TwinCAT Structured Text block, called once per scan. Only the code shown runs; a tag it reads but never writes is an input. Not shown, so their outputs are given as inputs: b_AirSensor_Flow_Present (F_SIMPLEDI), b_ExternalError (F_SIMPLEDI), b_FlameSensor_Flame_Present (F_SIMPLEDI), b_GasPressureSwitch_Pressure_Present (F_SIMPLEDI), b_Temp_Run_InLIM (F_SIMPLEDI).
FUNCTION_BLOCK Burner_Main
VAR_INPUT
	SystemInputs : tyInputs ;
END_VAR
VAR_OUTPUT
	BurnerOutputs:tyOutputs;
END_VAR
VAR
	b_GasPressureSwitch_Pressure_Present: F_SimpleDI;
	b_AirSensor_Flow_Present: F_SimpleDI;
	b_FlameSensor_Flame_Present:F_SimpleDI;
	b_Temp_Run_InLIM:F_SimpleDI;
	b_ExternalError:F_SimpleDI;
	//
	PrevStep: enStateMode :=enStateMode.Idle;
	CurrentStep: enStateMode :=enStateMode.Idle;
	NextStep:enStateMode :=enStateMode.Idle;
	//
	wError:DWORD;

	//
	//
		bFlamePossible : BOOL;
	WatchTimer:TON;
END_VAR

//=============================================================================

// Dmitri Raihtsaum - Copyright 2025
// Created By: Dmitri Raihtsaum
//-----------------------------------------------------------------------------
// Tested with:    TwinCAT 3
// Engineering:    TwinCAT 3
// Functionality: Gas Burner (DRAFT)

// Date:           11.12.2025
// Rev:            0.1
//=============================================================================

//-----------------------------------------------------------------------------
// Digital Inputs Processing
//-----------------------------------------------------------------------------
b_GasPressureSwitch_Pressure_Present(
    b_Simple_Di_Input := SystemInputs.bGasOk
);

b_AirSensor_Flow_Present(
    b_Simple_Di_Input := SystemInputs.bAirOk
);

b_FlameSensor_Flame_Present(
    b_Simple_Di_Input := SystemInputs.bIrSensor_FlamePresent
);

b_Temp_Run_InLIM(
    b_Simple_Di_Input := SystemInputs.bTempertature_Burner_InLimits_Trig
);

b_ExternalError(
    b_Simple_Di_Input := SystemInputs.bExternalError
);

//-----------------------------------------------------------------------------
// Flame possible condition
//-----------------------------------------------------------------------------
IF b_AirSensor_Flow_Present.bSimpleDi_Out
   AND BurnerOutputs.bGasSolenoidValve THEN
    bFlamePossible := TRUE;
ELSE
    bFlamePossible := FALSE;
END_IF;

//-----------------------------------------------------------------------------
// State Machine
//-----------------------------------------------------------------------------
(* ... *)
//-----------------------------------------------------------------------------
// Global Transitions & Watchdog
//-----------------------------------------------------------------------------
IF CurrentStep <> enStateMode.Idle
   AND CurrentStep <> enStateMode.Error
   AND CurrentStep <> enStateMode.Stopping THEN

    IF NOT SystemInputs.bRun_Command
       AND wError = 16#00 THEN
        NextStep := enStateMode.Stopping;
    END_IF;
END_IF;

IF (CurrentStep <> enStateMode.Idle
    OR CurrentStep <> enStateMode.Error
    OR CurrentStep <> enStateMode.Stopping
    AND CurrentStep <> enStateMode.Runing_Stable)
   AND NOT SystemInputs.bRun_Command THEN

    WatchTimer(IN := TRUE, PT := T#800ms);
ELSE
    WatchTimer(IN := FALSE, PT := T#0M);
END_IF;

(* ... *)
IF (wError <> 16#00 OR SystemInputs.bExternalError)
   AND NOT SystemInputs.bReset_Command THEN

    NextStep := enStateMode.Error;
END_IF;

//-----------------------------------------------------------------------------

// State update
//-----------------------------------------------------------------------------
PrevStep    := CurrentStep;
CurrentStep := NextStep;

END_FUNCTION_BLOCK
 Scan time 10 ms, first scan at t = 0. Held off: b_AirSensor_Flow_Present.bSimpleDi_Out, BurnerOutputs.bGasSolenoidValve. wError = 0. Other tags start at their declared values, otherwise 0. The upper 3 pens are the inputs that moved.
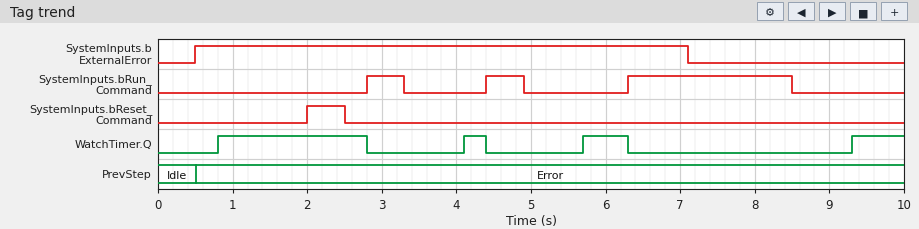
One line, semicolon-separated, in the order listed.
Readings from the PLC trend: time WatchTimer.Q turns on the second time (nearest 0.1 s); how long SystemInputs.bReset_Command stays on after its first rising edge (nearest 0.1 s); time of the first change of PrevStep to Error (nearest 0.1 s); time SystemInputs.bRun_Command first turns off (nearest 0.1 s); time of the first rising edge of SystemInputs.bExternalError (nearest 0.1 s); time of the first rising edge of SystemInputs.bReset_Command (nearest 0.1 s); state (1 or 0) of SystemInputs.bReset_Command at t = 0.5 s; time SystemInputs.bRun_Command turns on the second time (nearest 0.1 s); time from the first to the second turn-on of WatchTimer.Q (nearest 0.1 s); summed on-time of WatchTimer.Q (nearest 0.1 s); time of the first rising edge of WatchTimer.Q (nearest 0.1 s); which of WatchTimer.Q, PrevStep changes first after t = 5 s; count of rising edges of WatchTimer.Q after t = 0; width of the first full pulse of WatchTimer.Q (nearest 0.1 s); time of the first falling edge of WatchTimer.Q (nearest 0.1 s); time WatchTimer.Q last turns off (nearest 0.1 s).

4.1 s; 0.5 s; 0.5 s; 3.3 s; 0.5 s; 2.0 s; 0; 4.4 s; 3.3 s; 3.6 s; 0.8 s; WatchTimer.Q; 4; 2.0 s; 2.8 s; 6.3 s
